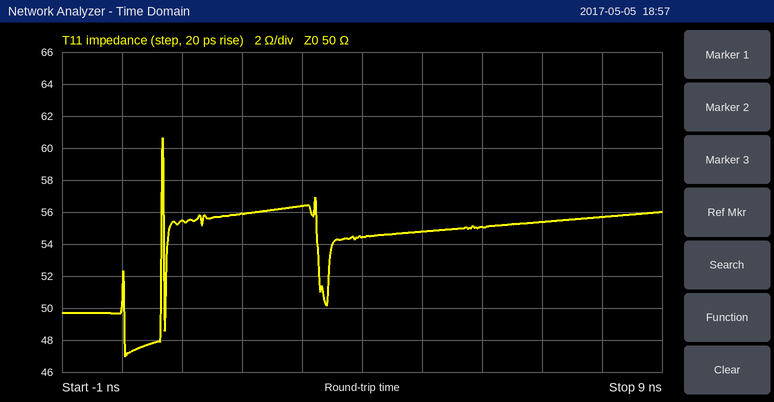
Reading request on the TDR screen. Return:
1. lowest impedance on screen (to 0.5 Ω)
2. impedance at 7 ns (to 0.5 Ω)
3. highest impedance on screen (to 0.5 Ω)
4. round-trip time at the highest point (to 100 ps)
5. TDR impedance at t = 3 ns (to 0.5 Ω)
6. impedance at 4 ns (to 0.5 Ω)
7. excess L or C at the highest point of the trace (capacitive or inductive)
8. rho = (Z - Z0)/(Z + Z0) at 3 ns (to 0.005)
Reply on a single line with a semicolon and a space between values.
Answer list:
47.0 Ω; 55.5 Ω; 60.5 Ω; 700 ps; 56.5 Ω; 54.5 Ω; inductive; +0.060
